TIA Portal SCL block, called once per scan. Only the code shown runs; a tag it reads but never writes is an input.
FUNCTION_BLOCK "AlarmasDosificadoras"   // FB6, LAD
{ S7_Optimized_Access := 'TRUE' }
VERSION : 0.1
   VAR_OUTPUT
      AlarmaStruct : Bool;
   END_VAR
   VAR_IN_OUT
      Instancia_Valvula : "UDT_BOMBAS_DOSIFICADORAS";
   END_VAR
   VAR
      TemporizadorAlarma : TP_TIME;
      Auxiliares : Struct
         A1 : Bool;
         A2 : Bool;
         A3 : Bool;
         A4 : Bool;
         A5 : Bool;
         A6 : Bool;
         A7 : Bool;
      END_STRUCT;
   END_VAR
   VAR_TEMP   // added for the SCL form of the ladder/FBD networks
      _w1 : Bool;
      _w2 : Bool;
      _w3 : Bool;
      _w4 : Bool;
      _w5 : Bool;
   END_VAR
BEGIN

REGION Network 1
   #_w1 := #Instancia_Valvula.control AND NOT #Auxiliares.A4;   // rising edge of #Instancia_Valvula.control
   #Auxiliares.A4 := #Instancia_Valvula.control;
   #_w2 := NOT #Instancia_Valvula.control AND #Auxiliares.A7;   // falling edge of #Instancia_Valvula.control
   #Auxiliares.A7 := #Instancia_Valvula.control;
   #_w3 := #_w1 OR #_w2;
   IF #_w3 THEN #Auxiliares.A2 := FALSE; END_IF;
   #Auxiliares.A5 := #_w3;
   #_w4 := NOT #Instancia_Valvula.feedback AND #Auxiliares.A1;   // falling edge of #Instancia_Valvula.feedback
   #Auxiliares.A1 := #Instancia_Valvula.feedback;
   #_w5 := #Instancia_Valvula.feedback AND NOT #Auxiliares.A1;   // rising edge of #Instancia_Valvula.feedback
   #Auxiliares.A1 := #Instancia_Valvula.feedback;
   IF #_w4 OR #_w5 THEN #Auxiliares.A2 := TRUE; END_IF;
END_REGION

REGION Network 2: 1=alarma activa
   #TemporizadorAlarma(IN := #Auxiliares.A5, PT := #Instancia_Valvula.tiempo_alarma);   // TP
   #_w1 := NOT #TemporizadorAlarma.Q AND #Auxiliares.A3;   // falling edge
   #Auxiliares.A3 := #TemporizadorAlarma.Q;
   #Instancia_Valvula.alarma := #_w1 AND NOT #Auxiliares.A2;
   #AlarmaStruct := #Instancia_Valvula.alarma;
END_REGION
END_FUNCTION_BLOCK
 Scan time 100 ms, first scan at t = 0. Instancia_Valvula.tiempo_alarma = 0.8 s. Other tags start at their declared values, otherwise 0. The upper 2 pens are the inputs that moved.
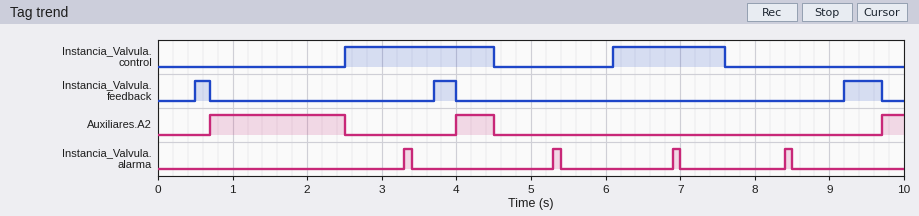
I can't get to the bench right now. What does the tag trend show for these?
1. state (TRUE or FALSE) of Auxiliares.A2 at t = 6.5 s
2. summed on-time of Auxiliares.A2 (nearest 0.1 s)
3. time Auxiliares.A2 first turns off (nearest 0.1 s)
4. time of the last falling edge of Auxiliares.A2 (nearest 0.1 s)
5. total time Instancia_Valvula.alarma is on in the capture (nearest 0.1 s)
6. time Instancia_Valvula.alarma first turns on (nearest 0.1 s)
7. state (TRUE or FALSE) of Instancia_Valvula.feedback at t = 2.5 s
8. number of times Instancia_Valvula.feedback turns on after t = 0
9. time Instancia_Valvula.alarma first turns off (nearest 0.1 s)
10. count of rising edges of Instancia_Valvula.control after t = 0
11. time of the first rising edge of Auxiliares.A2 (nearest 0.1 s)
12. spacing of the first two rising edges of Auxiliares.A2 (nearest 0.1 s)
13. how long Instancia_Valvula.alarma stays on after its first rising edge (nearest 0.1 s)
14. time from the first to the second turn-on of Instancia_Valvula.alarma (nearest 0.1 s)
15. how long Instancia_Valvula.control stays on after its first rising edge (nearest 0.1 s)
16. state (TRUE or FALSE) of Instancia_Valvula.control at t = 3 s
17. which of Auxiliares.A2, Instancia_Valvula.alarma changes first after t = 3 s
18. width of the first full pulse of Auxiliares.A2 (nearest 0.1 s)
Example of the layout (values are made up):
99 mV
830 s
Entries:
FALSE
2.6 s
2.5 s
4.5 s
0.4 s
3.3 s
FALSE
3
3.4 s
2
0.7 s
3.3 s
0.1 s
2.0 s
2.0 s
TRUE
Instancia_Valvula.alarma
1.8 s
